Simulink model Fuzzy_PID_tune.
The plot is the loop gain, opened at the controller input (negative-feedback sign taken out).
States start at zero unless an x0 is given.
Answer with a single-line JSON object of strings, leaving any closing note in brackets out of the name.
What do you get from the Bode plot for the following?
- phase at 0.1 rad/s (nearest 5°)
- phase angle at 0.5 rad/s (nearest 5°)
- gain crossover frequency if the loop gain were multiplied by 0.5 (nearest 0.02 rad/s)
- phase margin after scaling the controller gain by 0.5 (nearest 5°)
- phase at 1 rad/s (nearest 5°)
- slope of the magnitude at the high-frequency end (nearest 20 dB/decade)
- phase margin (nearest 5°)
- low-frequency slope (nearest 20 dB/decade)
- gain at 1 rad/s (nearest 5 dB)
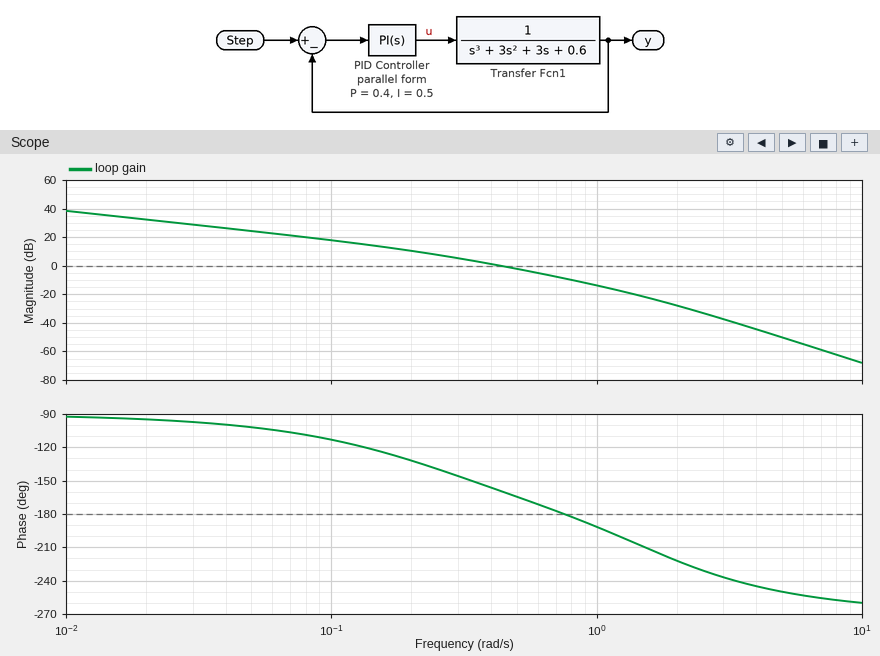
{"phase at 0.1 rad/s": "-115°", "phase angle at 0.5 rad/s": "-165°", "gain crossover frequency if the loop gain were multiplied by 0.5": "0.28 rad/s", "phase margin after scaling the controller gain by 0.5": "35°", "phase at 1 rad/s": "-190°", "slope of the magnitude at the high-frequency end": "-60 dB/decade", "phase margin": "20°", "low-frequency slope": "-20 dB/decade", "gain at 1 rad/s": "-15 dB"}
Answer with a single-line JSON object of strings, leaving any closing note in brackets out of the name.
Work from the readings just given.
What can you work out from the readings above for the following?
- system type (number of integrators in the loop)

{"system type": "1"}
